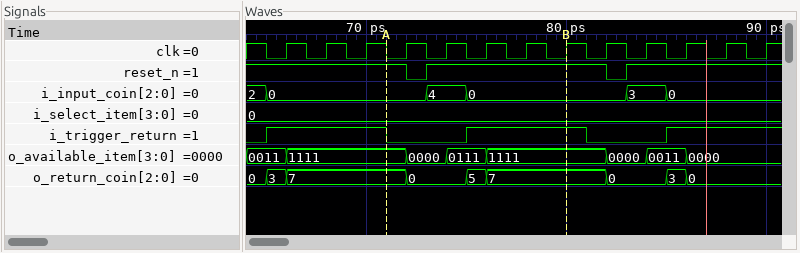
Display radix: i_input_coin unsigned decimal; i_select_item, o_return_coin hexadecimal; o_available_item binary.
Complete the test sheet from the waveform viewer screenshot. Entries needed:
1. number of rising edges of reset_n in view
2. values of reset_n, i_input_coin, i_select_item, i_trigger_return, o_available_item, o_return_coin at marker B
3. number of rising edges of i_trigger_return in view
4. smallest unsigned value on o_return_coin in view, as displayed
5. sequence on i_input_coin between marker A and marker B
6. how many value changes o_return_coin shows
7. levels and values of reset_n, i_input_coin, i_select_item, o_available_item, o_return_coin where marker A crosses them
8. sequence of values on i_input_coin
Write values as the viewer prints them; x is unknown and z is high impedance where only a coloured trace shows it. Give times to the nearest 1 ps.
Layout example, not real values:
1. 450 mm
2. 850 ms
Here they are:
1. 2
2. reset_n=1, i_input_coin=0, i_select_item=0, i_trigger_return=1, o_available_item=1111, o_return_coin=7
3. 3
4. 0
5. 0, 4, 0
6. 8
7. reset_n=1, i_input_coin=0, i_select_item=0, o_available_item=1111, o_return_coin=7
8. 2, 0, 4, 0, 3, 0
